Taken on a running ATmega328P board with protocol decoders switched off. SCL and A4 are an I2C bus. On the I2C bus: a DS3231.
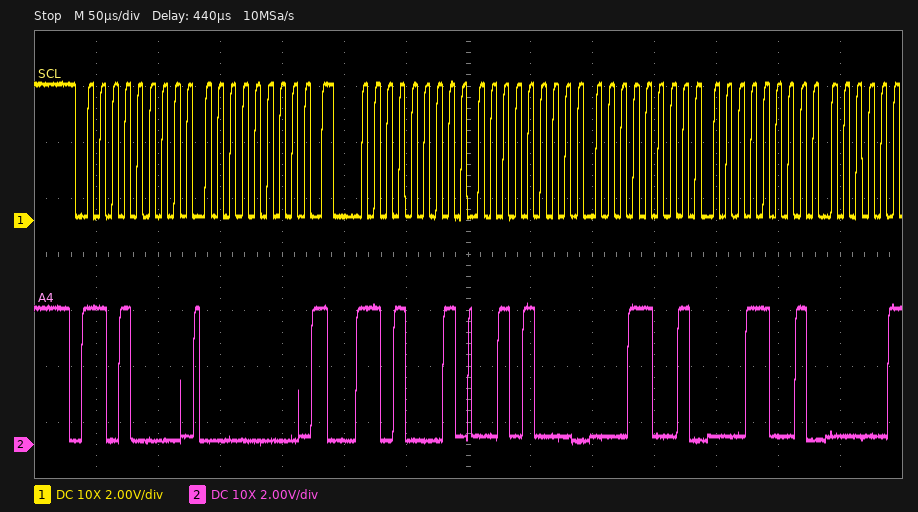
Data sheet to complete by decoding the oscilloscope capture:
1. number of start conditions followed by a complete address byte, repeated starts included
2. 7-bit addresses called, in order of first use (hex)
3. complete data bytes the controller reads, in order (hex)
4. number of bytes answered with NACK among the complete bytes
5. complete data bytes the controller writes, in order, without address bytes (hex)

2
0x68
28 19 19
0
00
